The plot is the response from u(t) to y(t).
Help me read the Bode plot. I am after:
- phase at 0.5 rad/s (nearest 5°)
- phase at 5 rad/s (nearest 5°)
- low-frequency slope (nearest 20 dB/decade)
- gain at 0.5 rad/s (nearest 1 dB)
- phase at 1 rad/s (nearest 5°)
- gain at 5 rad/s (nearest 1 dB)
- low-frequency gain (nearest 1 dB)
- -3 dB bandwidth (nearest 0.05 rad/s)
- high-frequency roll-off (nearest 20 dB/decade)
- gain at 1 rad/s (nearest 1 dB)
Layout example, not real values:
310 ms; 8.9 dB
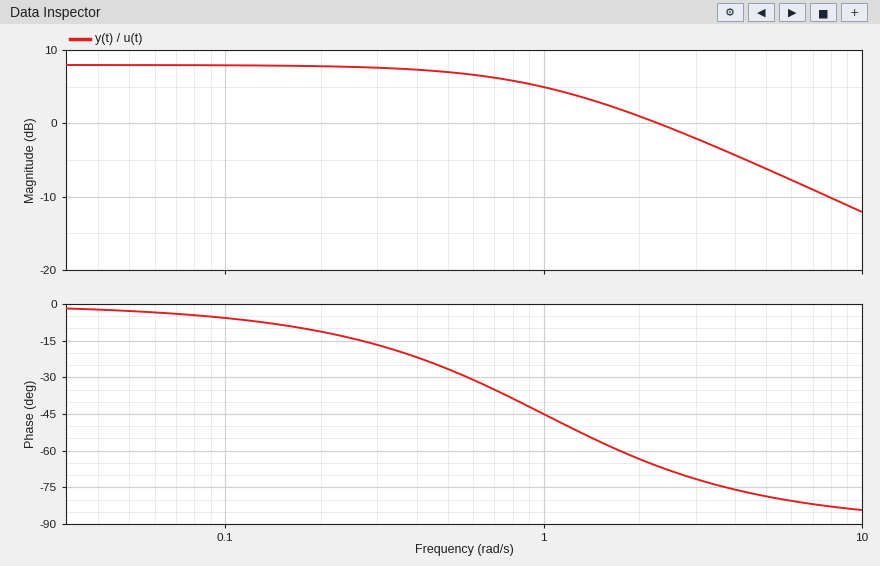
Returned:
-25°; -80°; 0 dB/decade; 7 dB; -45°; -6 dB; 8 dB; 1.00 rad/s; -20 dB/decade; 5 dB
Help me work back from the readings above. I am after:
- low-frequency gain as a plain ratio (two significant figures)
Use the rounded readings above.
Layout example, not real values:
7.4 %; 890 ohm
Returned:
2.5
